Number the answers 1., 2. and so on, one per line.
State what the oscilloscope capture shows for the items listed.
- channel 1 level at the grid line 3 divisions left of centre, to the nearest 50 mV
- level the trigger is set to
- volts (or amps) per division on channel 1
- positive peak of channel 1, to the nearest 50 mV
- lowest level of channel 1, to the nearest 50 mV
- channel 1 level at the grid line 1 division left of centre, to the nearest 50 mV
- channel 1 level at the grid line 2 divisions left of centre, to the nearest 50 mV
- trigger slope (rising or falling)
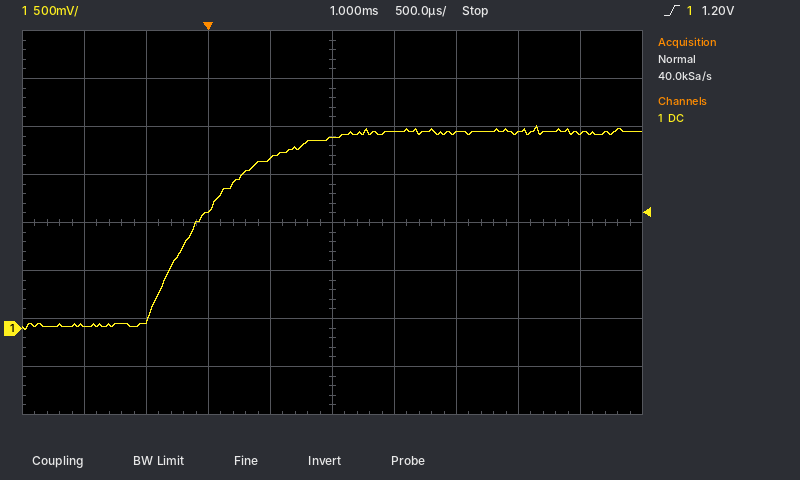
1. 100 mV
2. 1.20 V
3. 500 mV
4. 2.10 V
5. 0 mV
6. 1.75 V
7. 1.20 V
8. rising
